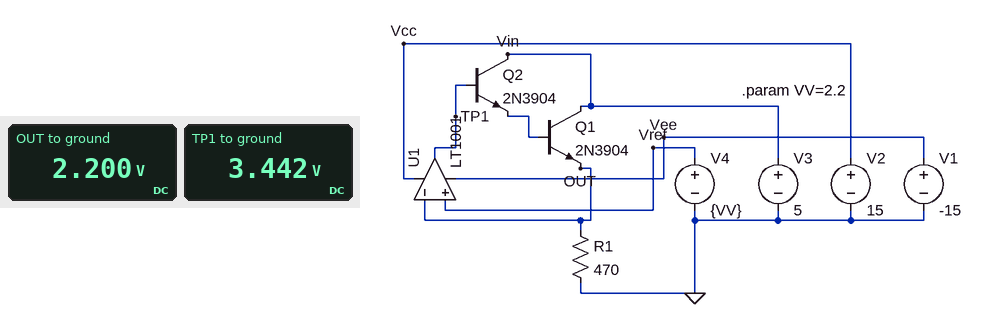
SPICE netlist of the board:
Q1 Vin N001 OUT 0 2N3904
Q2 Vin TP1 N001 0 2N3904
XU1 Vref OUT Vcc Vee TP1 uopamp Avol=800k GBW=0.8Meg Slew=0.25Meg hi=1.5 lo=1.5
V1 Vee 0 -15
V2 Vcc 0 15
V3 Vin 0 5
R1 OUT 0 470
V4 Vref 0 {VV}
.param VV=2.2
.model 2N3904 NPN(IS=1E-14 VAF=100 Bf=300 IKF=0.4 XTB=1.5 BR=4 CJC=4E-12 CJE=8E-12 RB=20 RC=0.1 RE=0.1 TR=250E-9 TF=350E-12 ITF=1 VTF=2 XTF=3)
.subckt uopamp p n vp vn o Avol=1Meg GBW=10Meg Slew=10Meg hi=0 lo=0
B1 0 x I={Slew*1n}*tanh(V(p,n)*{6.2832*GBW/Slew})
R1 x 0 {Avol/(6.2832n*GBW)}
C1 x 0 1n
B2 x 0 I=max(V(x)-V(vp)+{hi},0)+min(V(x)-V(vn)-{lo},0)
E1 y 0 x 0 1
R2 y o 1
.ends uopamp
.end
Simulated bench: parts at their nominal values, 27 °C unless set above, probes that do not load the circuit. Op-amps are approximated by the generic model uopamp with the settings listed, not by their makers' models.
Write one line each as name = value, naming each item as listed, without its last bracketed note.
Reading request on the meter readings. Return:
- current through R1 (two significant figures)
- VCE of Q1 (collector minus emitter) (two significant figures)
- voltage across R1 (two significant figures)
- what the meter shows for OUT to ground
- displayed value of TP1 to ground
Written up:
current through R1 = 4.7 mA
VCE of Q1 (collector minus emitter) = 2.8 V
voltage across R1 = 2.2 V
what the meter shows for OUT to ground = 2.200 V
displayed value of TP1 to ground = 3.442 V
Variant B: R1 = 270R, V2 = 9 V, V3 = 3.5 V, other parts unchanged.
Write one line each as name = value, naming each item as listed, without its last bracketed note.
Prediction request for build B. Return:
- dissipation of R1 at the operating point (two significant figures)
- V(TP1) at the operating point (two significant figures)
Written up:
dissipation of R1 at the operating point = 18 mW
V(TP1) at the operating point = 3.5 V
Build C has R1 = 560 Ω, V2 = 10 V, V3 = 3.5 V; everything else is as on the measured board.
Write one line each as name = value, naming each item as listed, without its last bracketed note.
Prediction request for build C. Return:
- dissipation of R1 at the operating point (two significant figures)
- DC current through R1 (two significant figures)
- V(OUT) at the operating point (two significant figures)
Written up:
dissipation of R1 at the operating point = 8.6 mW
DC current through R1 = 3.9 mA
V(OUT) at the operating point = 2.2 V
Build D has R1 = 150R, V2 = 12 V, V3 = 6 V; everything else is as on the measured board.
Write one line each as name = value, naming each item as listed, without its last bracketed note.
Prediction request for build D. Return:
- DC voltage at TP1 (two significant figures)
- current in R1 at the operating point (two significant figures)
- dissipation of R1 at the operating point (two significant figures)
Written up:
DC voltage at TP1 = 3.5 V
current in R1 at the operating point = 15 mA
dissipation of R1 at the operating point = 32 mW
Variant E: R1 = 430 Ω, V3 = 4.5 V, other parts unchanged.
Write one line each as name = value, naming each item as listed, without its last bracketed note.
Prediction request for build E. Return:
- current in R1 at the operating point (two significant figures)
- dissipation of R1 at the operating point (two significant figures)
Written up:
current in R1 at the operating point = 5.1 mA
dissipation of R1 at the operating point = 11 mW
